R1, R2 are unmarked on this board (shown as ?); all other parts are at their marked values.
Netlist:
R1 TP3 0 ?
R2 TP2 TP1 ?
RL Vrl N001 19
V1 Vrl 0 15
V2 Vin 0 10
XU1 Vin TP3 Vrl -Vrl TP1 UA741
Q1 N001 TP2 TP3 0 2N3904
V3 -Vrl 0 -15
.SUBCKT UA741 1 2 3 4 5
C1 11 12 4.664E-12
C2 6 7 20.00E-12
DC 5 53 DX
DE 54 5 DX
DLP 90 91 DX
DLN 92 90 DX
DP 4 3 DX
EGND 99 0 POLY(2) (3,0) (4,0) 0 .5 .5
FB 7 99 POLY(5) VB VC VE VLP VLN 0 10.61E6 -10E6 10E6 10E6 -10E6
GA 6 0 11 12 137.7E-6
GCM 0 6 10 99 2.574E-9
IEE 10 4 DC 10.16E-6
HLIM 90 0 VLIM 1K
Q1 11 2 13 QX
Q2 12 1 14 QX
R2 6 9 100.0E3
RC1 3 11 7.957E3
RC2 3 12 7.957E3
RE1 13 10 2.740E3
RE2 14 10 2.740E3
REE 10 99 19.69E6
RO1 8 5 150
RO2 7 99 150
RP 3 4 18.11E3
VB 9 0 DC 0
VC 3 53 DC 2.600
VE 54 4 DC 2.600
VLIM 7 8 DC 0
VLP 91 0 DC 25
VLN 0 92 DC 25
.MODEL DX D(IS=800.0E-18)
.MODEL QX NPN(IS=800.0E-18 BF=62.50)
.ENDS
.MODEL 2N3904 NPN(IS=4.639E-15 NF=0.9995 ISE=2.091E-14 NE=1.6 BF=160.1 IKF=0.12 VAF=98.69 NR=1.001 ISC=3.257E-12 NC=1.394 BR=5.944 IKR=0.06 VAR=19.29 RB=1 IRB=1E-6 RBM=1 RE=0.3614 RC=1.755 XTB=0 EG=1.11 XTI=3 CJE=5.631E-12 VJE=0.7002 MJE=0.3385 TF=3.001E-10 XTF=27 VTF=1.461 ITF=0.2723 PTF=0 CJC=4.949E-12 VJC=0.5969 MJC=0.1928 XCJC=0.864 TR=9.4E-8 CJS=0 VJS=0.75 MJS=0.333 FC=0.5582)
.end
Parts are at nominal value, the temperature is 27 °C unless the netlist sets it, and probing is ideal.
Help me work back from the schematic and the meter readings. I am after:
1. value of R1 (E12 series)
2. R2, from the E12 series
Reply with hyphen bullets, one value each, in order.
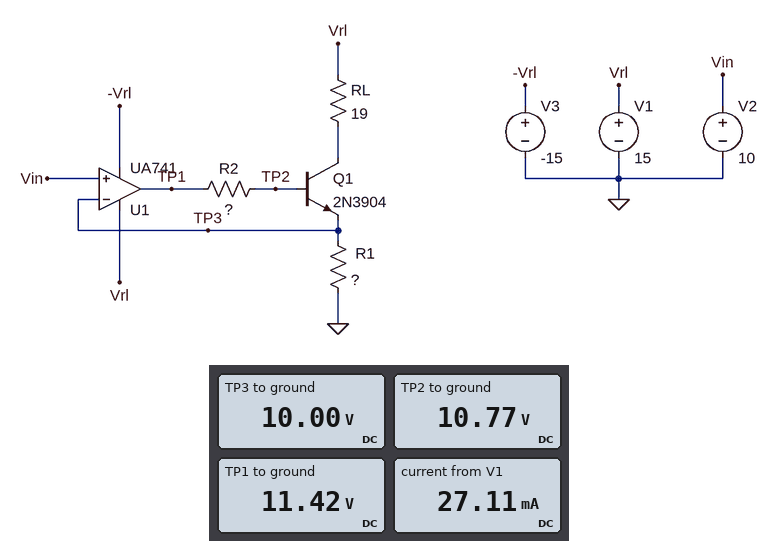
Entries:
- 390 Ω
- 3.3 kΩ
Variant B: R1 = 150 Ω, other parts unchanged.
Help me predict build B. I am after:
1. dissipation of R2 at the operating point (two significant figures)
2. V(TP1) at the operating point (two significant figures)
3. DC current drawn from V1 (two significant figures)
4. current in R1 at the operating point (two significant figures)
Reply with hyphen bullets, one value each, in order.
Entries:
- 1.4 mW
- 13 V
- 68 mA
- 67 mA
